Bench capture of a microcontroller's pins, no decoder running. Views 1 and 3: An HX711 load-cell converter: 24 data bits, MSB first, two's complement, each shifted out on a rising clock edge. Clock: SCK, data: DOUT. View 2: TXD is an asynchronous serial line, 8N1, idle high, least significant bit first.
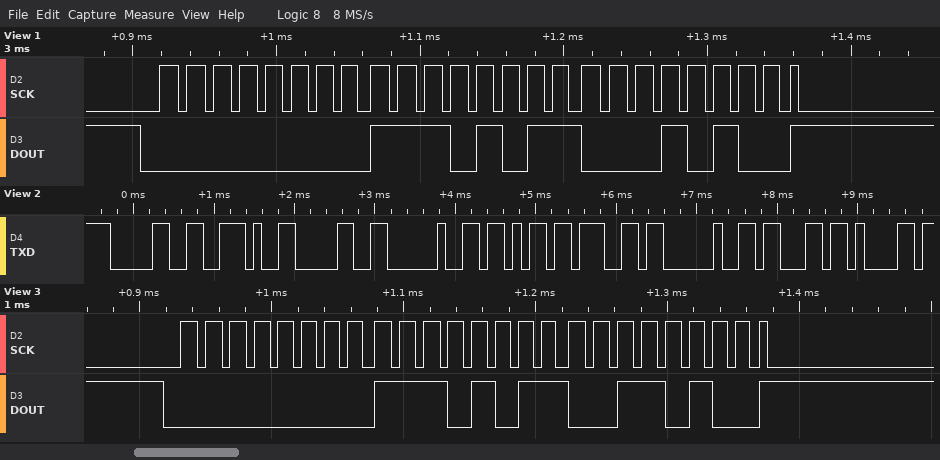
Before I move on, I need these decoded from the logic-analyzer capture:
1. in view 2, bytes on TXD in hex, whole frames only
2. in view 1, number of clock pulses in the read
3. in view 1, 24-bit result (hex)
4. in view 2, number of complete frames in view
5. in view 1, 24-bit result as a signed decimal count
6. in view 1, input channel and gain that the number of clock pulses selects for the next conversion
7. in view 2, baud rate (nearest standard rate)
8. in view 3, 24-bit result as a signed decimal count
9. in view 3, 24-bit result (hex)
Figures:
30 2E 30 20 6B 67 20 63 61
25
0x00EB14
9
60180
channel A, gain 128
9600 baud
60212
0x00EB34
